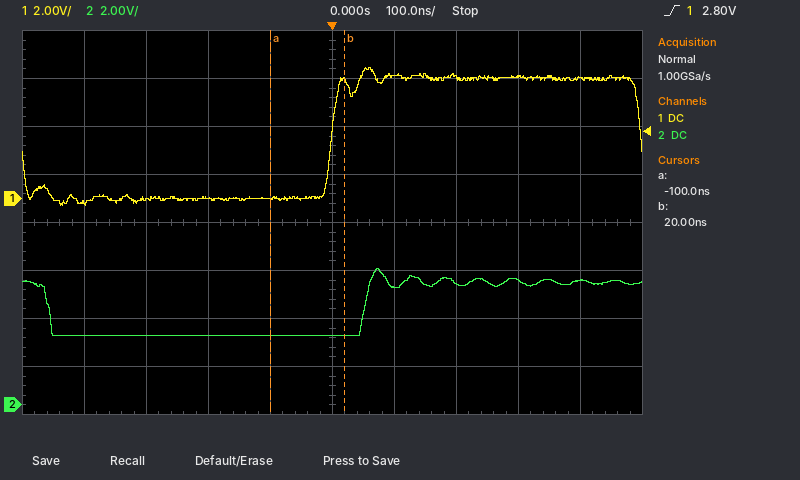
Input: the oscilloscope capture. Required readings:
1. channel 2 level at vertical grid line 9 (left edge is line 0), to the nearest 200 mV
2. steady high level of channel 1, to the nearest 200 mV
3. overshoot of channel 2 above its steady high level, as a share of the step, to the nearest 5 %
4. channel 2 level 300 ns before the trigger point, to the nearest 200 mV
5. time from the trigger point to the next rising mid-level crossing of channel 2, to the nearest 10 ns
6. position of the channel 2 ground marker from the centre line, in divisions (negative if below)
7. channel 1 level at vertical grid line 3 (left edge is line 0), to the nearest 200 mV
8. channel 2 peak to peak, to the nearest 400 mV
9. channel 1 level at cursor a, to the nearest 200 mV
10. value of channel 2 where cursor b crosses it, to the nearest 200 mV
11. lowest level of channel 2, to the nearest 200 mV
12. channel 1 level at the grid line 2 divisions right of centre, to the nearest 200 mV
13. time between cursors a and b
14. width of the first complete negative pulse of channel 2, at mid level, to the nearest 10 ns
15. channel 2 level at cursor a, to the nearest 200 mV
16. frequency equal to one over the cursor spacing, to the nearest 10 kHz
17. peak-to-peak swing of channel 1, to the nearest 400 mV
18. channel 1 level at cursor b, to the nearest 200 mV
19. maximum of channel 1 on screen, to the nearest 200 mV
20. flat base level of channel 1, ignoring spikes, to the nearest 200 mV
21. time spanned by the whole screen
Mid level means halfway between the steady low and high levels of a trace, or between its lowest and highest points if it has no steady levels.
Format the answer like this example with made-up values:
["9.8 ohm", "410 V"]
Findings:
["5.2 V", "5.0 V", "25 %", "2.8 V", "50 ns", "-3.8 div", "0.0 V", "2.8 V", "0.0 V", "2.8 V", "2.8 V", "5.0 V", "120 ns", "510 ns", "2.8 V", "8.33 MHz", "5.6 V", "4.8 V", "5.4 V", "0.0 V", "1 µs"]
